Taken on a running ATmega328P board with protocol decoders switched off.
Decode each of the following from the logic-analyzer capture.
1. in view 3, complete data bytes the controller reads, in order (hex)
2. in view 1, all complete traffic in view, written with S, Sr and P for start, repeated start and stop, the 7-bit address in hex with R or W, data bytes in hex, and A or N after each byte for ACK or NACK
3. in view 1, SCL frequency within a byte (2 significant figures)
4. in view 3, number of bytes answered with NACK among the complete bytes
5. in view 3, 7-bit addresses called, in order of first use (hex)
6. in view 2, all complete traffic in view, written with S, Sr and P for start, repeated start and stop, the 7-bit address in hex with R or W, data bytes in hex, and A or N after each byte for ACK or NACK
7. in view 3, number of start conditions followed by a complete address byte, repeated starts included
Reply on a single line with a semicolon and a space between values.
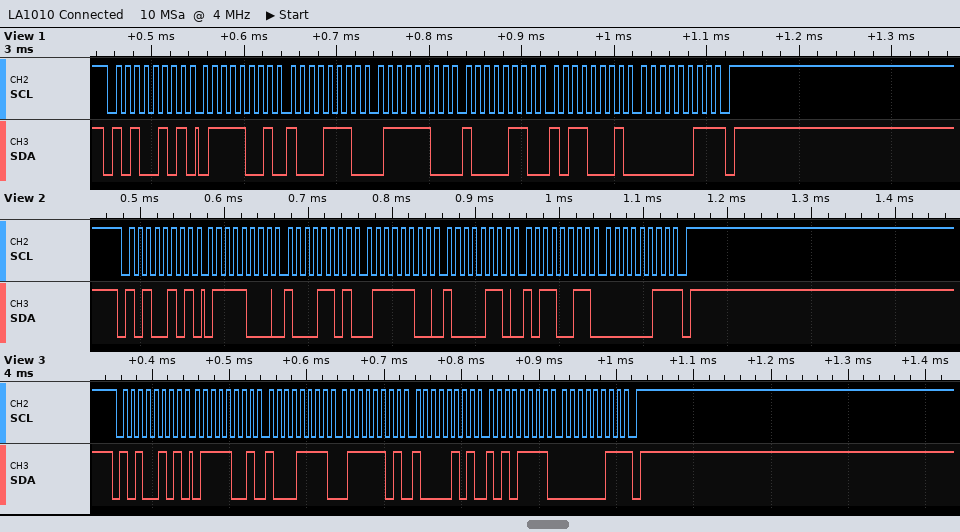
79 8F 7D 85 AF 03; S 52R A 79 A 8E A 7C A 86 A B1 A 03 N P; 100 kHz; 1; 0x52; S 52R A 78 A 8D A 7C A 86 A B3 A 03 N P; 1
